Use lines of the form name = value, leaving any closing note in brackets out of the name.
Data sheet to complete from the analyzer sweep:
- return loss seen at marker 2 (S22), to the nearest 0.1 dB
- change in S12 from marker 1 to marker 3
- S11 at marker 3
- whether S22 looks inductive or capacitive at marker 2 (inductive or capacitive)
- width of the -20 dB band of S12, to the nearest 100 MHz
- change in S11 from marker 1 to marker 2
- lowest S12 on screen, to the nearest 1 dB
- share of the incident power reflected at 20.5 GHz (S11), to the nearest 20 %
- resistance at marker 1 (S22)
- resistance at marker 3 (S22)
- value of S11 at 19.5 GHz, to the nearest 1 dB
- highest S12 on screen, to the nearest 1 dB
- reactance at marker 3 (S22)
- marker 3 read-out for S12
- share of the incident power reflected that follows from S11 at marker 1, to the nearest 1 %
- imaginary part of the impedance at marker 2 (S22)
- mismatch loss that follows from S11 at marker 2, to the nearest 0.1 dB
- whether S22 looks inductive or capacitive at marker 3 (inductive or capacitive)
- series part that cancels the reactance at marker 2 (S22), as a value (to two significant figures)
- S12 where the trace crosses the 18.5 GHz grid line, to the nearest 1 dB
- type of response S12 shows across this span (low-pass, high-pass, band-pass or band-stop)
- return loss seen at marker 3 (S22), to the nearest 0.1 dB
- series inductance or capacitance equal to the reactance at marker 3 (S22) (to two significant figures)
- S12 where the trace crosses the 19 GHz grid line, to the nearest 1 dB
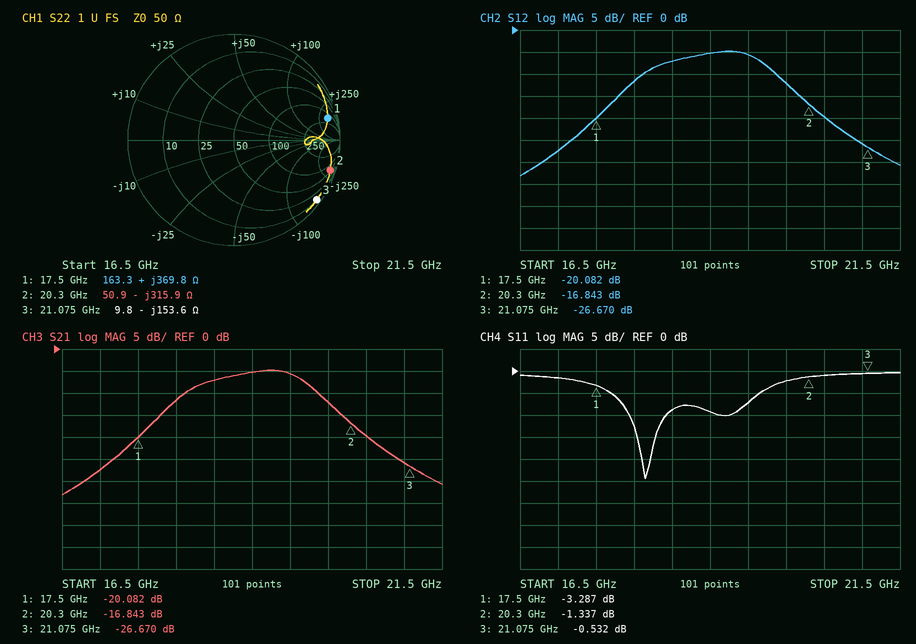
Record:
return loss seen at marker 2 (S22), to the nearest 0.1 dB = 0.4 dB
change in S12 from marker 1 to marker 3 = -6.588 dB
S11 at marker 3 = -0.532 dB
whether S22 looks inductive or capacitive at marker 2 = capacitive
width of the -20 dB band of S12, to the nearest 100 MHz = 3.7 GHz
change in S11 from marker 1 to marker 2 = 1.950 dB
lowest S12 on screen, to the nearest 1 dB = -33 dB
share of the incident power reflected at 20.5 GHz (S11), to the nearest 20 % = 80 %
resistance at marker 1 = 163.3 Ω
resistance at marker 3 = 9.8 Ω
value of S11 at 19.5 GHz, to the nearest 1 dB = -7 dB
highest S12 on screen, to the nearest 1 dB = -5 dB
reactance at marker 3 = -153.6 Ω
marker 3 read-out for S12 = -26.670 dB
share of the incident power reflected that follows from S11 at marker 1, to the nearest 1 % = 47 %
imaginary part of the impedance at marker 2 = -315.9 Ω
mismatch loss that follows from S11 at marker 2, to the nearest 0.1 dB = 5.8 dB
whether S22 looks inductive or capacitive at marker 3 = capacitive
series part that cancels the reactance at marker 2 (S22), as a value = 2.5 nH
S12 where the trace crosses the 18.5 GHz grid line, to the nearest 1 dB = -7 dB
type of response S12 shows across this span = band-pass
return loss seen at marker 3 (S22), to the nearest 0.1 dB = 0.3 dB
series inductance or capacitance equal to the reactance at marker 3 (S22) = 49 fF
S12 where the trace crosses the 19 GHz grid line, to the nearest 1 dB = -5 dB
